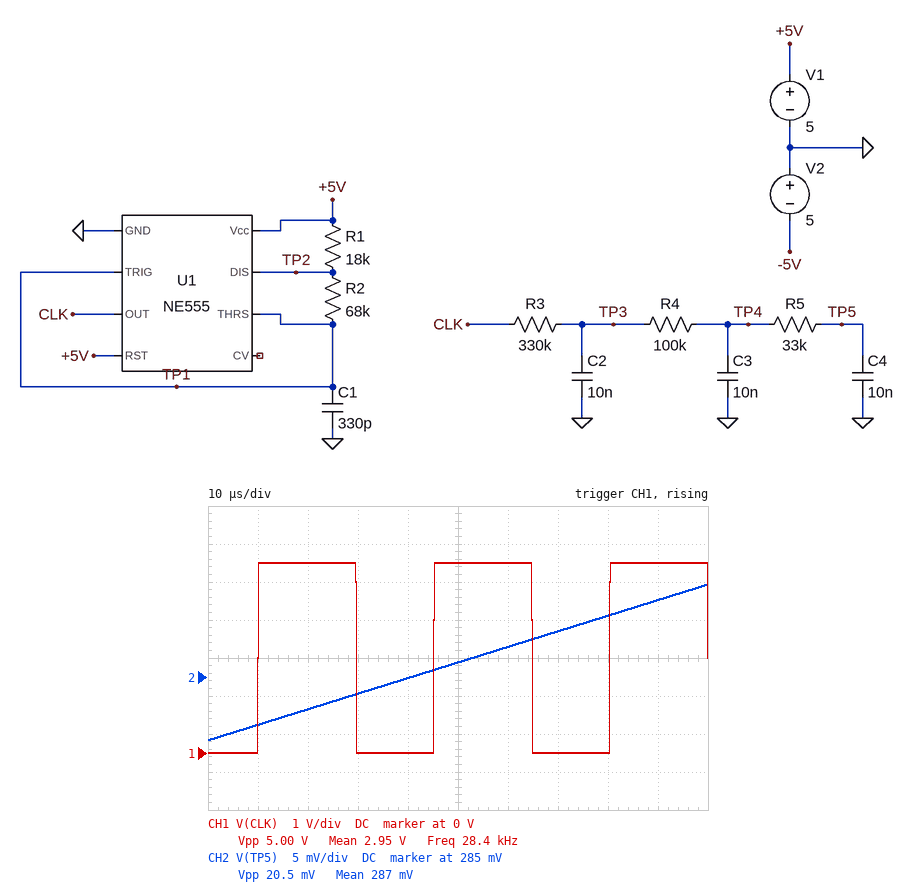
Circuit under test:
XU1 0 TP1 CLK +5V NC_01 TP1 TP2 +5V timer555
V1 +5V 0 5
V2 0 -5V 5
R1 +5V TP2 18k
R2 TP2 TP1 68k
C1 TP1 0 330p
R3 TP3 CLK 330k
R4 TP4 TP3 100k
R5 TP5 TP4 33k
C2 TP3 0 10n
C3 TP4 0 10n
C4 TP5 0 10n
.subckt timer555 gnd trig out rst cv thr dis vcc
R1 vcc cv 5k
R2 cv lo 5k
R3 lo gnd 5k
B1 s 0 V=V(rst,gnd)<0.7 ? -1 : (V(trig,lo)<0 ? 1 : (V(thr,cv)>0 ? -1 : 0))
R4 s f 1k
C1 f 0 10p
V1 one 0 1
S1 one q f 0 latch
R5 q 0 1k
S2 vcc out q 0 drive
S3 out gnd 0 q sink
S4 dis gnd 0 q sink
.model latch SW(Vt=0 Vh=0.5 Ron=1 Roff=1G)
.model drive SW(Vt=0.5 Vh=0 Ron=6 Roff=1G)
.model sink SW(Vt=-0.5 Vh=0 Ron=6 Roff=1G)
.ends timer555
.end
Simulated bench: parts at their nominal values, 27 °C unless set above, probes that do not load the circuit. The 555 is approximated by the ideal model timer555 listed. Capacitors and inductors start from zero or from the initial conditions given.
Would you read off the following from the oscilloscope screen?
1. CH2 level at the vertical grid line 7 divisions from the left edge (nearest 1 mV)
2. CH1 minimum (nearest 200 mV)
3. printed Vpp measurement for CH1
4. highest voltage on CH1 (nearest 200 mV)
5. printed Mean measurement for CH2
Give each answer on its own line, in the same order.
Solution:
291 mV
0 V
5.00 V
5.0 V
287 mV
